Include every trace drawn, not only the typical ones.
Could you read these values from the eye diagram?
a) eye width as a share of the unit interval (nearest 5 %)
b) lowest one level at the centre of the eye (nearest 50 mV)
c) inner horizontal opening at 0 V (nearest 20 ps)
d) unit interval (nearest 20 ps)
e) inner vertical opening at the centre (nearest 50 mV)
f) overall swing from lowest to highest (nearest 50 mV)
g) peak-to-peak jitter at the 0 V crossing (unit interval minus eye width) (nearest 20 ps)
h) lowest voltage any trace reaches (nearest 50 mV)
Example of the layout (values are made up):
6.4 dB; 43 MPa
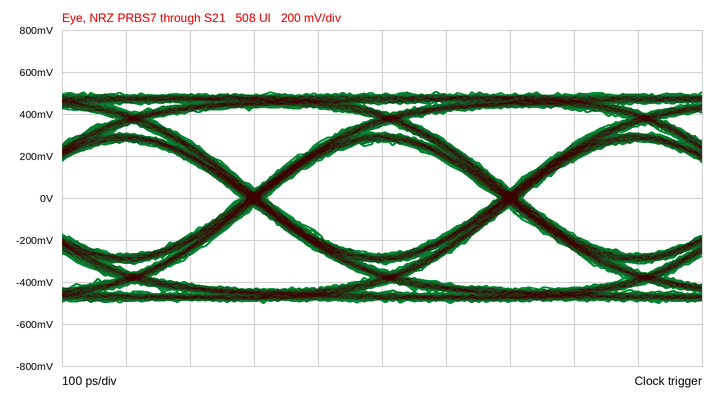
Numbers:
90 %; 250 mV; 360 ps; 400 ps; 550 mV; 1.00 V; 40 ps; -500 mV
